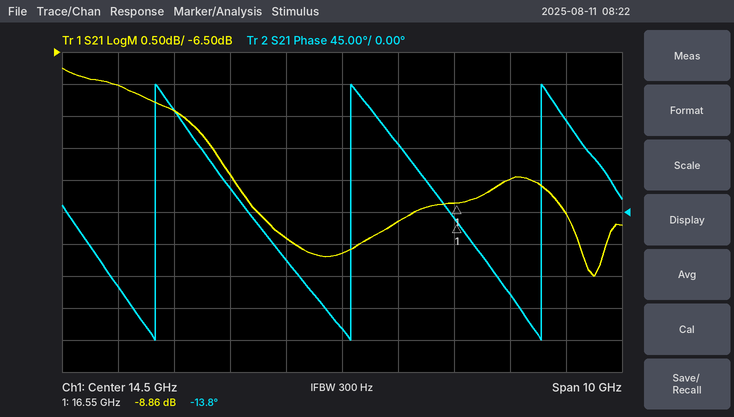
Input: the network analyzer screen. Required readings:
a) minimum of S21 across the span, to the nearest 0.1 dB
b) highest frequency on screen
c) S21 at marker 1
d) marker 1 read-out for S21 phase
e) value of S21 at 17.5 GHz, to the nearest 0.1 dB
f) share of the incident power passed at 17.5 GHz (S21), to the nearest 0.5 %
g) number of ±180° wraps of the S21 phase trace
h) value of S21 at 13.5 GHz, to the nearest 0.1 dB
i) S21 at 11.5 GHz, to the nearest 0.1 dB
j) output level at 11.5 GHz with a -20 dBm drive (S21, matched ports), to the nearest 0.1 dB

-10.0 dB
19.5 GHz
-8.86 dB
-13.8°
-8.5 dB
14.0 %
3
-9.4 dB
-7.4 dB
-27.4 dBm
